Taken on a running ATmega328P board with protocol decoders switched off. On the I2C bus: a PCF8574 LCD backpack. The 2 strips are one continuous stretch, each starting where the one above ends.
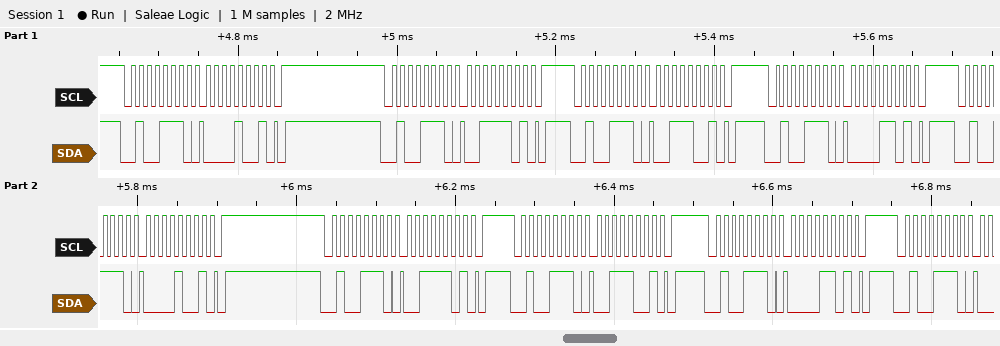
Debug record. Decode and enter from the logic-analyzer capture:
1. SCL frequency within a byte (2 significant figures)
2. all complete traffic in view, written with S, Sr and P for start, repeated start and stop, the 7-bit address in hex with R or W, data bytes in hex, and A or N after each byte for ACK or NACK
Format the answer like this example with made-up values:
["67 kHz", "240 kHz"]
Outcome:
["100 kHz", "S 27W A 09 A P S 27W A 3D A P S 27W A 39 A P S 27W A 0D A P S 27W A 09 A P S 27W A 3D A P S 27W A 39 A P S 27W A 0D A P S 27W A"]
